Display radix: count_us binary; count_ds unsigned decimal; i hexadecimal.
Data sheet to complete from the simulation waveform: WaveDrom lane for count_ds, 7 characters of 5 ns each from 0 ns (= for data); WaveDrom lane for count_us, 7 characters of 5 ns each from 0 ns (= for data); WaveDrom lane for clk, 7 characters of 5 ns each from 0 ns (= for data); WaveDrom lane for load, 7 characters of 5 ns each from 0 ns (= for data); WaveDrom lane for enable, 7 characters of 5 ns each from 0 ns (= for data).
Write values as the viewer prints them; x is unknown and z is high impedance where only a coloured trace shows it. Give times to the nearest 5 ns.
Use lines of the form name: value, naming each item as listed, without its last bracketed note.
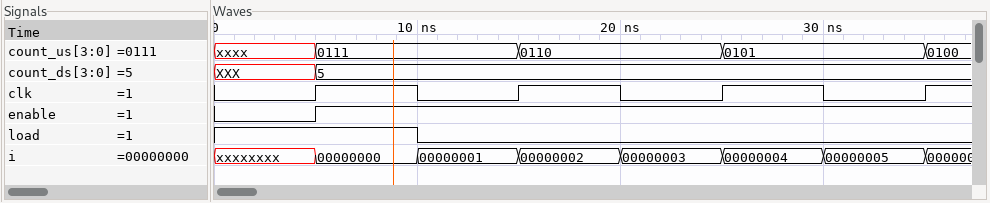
WaveDrom lane for count_ds, 7 characters of 5 ns each from 0 ns: {name: 'count_ds', wave: 'x=.....', data: '5'}
WaveDrom lane for count_us, 7 characters of 5 ns each from 0 ns: {name: 'count_us', wave: 'x=.=.=.', data: '0111 0110 0101'}
WaveDrom lane for clk, 7 characters of 5 ns each from 0 ns: {name: 'clk', wave: '0101010'}
WaveDrom lane for load, 7 characters of 5 ns each from 0 ns: {name: 'load', wave: '1.0....'}
WaveDrom lane for enable, 7 characters of 5 ns each from 0 ns: {name: 'enable', wave: '01.....'}
